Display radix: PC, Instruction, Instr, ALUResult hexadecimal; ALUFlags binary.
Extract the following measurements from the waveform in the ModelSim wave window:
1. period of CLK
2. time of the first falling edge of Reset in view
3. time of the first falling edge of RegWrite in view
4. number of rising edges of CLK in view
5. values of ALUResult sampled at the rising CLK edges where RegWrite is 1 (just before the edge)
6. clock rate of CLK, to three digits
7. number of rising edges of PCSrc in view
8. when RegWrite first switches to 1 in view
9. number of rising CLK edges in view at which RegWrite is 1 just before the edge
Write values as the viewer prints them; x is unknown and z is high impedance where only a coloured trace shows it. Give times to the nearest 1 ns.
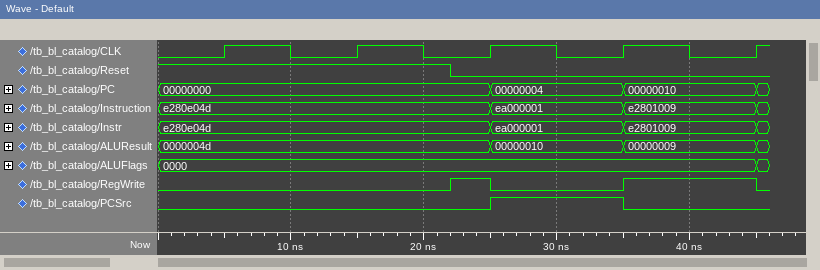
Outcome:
10 ns
22 ns
25 ns
5
0000004d, 00000009
100 MHz
1
22 ns
2
